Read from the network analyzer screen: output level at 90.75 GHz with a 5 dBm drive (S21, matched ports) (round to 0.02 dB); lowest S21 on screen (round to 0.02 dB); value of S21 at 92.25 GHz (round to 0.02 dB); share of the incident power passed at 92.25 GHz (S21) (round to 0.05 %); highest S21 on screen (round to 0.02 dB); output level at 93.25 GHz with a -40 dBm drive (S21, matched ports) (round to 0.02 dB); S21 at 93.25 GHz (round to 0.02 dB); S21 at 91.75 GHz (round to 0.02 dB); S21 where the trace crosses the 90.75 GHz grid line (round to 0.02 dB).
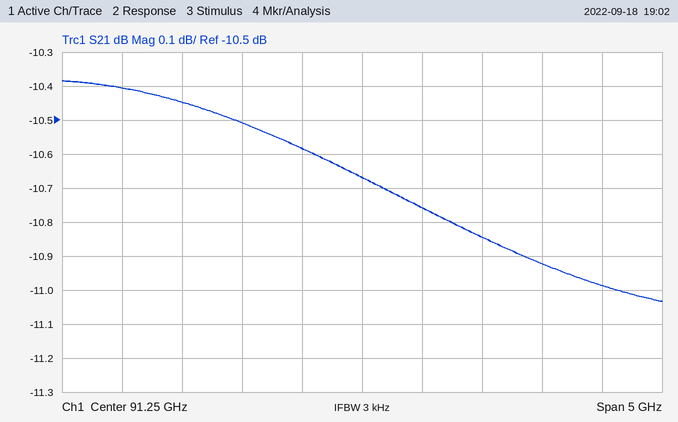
-5.58 dBm
-11.04 dB
-10.84 dB
8.25 %
-10.38 dB
-50.98 dBm
-10.98 dB
-10.76 dB
-10.58 dB
